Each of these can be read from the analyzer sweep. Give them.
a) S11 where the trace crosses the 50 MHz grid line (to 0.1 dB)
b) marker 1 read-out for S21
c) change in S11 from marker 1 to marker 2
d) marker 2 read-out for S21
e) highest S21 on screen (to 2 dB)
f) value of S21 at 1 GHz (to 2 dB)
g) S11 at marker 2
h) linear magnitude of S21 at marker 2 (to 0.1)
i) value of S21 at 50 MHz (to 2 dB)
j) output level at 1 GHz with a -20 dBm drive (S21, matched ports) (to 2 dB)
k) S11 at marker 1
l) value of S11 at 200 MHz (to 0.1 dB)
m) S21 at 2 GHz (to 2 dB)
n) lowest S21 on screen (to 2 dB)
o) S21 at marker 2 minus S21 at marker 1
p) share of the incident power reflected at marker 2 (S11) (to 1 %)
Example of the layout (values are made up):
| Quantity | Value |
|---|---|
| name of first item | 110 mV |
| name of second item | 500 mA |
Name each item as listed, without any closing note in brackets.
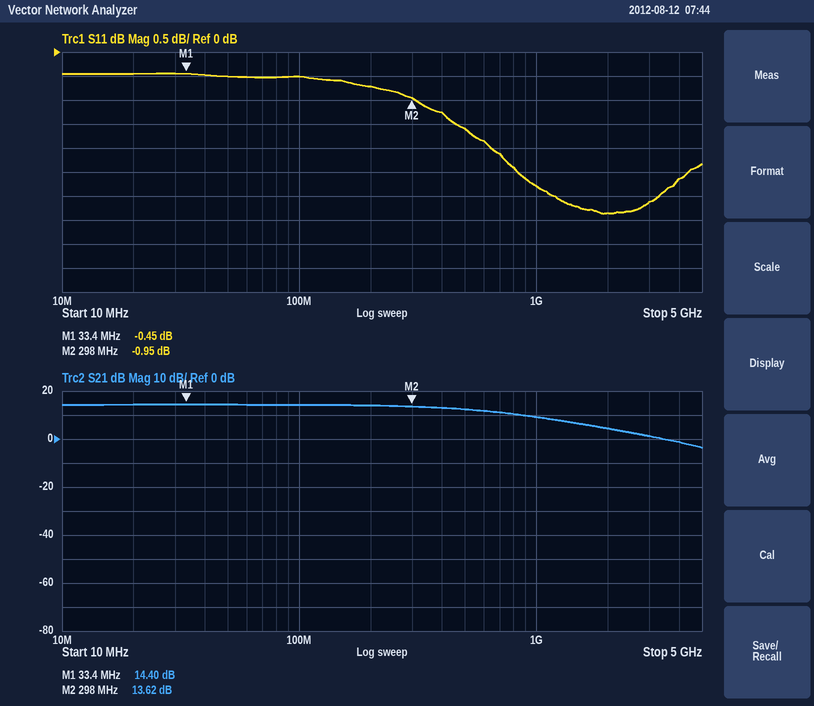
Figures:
| Quantity | Value |
|---|---|
| S11 where the trace crosses the 50 MHz grid line | -0.5 dB |
| marker 1 read-out for S21 | 14.40 dB |
| change in S11 from marker 1 to marker 2 | -0.50 dB |
| marker 2 read-out for S21 | 13.62 dB |
| highest S21 on screen | 14 dB |
| value of S21 at 1 GHz | 10 dB |
| S11 at marker 2 | -0.95 dB |
| linear magnitude of S21 at marker 2 | 4.8 |
| value of S21 at 50 MHz | 14 dB |
| output level at 1 GHz with a -20 dBm drive (S21, matched ports) | -10 dBm |
| S11 at marker 1 | -0.45 dB |
| value of S11 at 200 MHz | -0.7 dB |
| S21 at 2 GHz | 4 dB |
| lowest S21 on screen | -4 dB |
| S21 at marker 2 minus S21 at marker 1 | -0.78 dB |
| share of the incident power reflected at marker 2 (S11) | 80 % |
